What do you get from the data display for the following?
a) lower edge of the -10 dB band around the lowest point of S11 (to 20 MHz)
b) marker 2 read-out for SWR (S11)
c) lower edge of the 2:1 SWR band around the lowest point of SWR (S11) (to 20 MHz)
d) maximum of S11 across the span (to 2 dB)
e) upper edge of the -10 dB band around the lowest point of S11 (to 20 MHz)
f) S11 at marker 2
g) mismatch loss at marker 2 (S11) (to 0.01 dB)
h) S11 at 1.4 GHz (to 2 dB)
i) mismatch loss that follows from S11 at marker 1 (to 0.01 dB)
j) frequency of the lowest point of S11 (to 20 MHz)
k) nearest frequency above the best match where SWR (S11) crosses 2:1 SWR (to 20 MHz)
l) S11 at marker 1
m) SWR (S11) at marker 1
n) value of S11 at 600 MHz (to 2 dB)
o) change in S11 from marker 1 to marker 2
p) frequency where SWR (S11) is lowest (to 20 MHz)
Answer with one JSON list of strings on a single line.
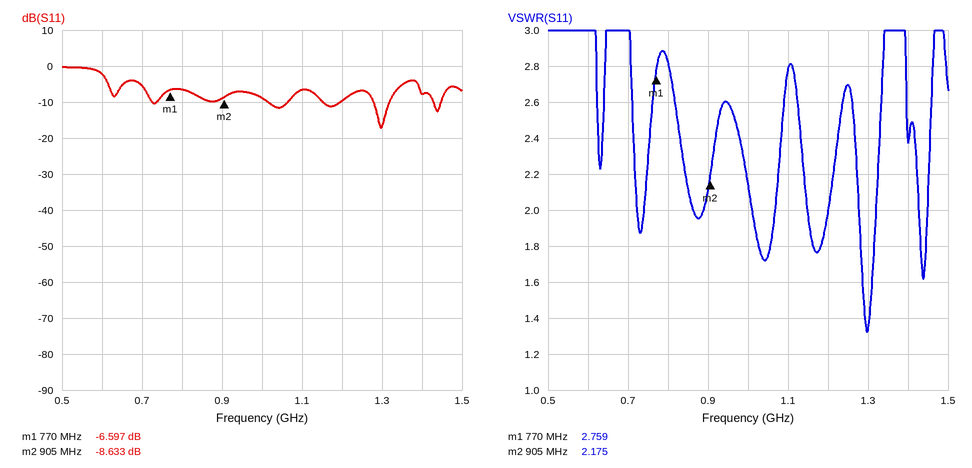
["1.28 GHz", "2.175", "1.28 GHz", "0 dB", "1.32 GHz", "-8.633 dB", "0.64 dB", "-8 dB", "1.07 dB", "1.30 GHz", "1.32 GHz", "-6.597 dB", "2.759", "-2 dB", "-2.036 dB", "1.30 GHz"]
